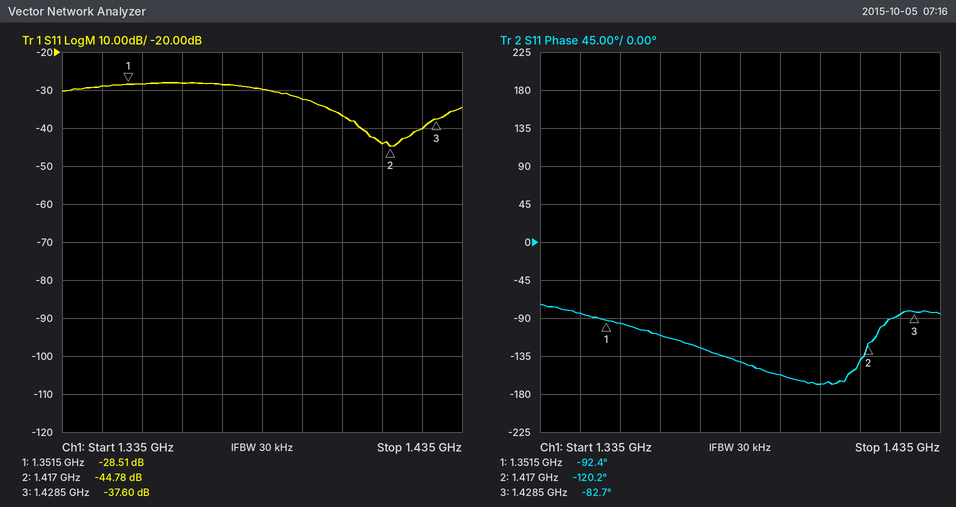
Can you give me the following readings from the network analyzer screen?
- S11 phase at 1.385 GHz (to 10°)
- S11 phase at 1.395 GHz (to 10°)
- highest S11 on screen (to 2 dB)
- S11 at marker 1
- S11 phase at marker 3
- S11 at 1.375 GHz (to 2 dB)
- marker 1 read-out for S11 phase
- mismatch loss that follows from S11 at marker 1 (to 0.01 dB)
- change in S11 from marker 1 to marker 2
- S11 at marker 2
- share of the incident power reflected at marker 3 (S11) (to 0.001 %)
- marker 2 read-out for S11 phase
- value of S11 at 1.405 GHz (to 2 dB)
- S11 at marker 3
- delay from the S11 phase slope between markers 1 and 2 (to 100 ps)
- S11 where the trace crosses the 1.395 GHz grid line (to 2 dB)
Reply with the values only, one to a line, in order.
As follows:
-140°
-160°
-28 dB
-28.51 dB
-82.7°
-28 dB
-92.4°
0.01 dB
-16.27 dB
-44.78 dB
0.017 %
-120.2°
-36 dB
-37.60 dB
1.2 ns
-32 dB
